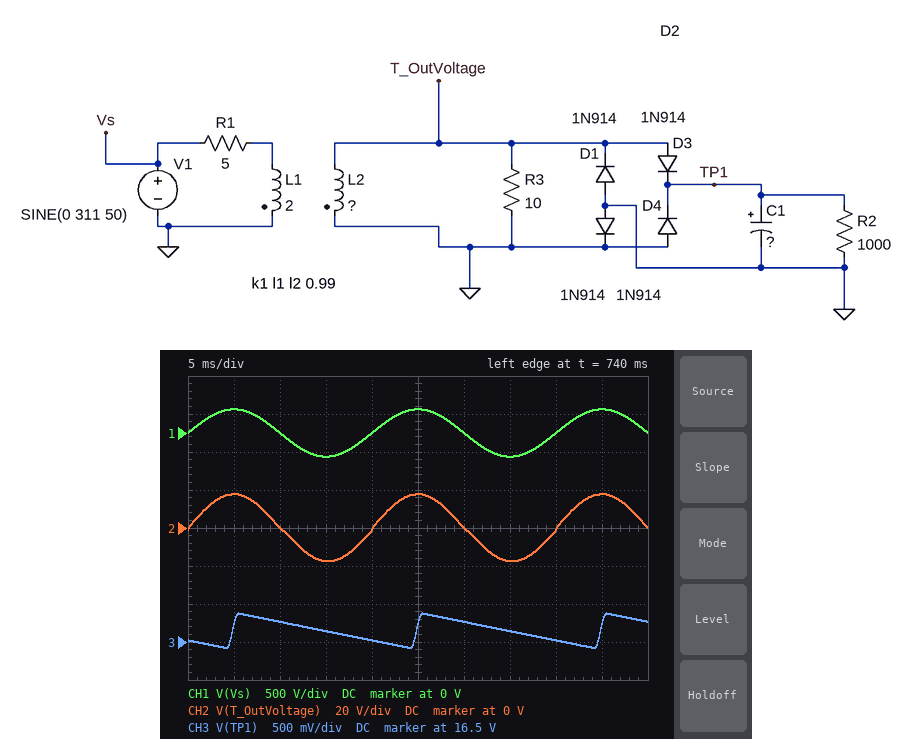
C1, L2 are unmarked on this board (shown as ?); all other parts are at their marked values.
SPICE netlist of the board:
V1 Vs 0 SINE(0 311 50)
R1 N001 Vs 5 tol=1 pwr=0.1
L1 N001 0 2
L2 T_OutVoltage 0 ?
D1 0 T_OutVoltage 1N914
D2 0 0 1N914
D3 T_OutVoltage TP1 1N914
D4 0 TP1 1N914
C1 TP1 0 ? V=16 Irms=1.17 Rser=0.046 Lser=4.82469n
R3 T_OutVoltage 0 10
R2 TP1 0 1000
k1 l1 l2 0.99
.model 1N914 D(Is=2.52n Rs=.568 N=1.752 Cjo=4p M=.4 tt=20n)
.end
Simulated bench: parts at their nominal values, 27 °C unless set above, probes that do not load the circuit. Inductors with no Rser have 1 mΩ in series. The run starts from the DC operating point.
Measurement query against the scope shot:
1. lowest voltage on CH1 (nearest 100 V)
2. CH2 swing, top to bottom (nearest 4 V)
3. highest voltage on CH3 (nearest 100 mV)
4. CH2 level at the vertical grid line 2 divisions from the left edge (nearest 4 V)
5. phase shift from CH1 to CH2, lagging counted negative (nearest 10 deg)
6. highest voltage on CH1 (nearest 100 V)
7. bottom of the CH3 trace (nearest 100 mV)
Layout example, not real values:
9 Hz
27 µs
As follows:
-300 V
36 V
16.9 V
0 V
0 deg
300 V
16.4 V
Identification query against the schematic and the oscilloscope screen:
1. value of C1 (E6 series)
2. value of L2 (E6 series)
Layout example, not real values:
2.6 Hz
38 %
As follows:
680 µF
6.8 mH
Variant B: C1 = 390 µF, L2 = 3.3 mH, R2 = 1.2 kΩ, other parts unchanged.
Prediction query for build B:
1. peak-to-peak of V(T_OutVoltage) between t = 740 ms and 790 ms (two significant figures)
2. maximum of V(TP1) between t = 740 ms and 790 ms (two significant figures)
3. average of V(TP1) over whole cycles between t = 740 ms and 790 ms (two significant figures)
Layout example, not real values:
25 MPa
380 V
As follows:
25 V
12 V
11 V
